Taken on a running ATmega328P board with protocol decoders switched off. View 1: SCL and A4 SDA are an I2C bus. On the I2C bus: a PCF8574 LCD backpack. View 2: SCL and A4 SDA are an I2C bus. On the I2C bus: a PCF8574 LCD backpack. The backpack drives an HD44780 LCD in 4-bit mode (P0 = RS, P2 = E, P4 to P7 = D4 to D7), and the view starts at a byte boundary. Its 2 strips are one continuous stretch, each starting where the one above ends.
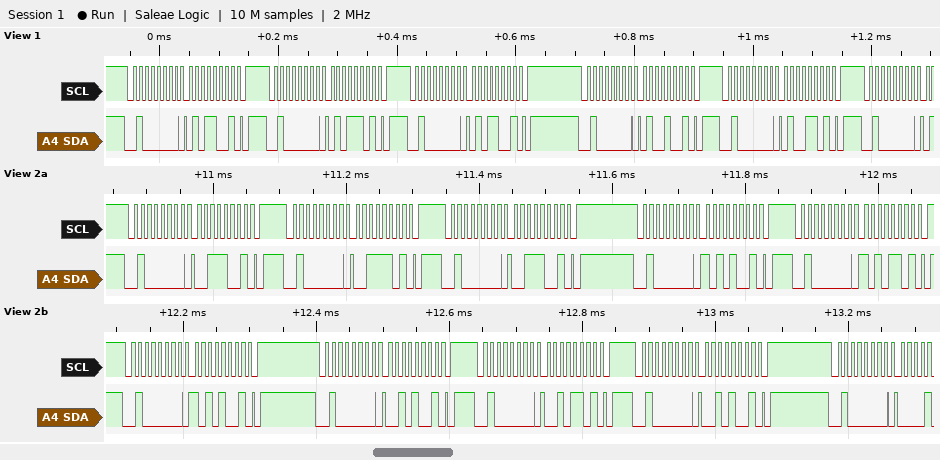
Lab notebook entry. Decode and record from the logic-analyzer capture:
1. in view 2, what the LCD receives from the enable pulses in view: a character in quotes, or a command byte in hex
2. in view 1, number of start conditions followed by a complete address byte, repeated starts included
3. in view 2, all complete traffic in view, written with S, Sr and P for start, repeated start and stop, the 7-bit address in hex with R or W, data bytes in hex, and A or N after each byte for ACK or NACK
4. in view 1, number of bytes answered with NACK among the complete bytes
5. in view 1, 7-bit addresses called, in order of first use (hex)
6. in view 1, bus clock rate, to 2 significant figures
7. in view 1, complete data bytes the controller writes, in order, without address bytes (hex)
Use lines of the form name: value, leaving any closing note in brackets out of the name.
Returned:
in view 2, what the LCD receives from the enable pulses in view: a character in quotes, or a command byte in hex: ':'
in view 1, number of start conditions followed by a complete address byte, repeated starts included: 6
in view 2, all complete traffic in view, written with S, Sr and P for start, repeated start and stop, the 7-bit address in hex with R or W, data bytes in hex, and A or N after each byte for ACK or NACK: S 20W A 39 A P S 20W A 3D A P S 20W A 39 A P S 20W A A9 A P S 20W A AD A P S 20W A A9 A P S 20W A 29 A P S 20W A 2D A P S 20W A 29 A P S 20W A
in view 1, number of bytes answered with NACK among the complete bytes: 0
in view 1, 7-bit addresses called, in order of first use: 0x20
in view 1, bus clock rate, to 2 significant figures: 100 kHz
in view 1, complete data bytes the controller writes, in order, without address bytes: 59 5D 59 49 4D
